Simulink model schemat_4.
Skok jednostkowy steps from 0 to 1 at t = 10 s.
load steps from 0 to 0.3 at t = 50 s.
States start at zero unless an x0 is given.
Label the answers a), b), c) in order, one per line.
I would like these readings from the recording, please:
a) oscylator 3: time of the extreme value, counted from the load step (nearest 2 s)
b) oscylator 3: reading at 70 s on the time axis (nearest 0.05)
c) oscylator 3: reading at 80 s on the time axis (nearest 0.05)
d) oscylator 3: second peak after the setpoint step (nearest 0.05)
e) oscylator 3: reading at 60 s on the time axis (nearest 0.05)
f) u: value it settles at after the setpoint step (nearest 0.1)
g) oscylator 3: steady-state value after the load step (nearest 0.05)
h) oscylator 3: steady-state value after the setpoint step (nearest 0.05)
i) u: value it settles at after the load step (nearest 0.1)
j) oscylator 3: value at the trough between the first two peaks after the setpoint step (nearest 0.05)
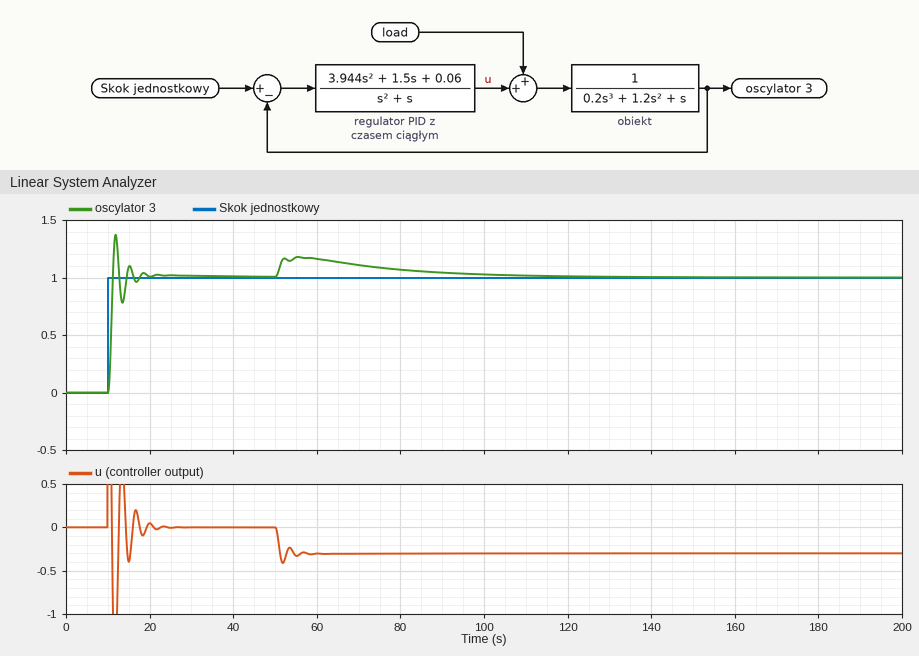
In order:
a) 6 s
b) 1.10
c) 1.05
d) 1.10
e) 1.15
f) 0.0
g) 1.00
h) 1.00
i) -0.3
j) 0.80
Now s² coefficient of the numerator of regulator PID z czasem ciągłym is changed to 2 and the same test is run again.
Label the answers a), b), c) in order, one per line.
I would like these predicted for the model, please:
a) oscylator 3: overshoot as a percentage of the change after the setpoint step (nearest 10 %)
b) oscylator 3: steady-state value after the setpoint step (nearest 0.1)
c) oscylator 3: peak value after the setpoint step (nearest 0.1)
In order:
a) 40 %
b) 1.0
c) 1.4
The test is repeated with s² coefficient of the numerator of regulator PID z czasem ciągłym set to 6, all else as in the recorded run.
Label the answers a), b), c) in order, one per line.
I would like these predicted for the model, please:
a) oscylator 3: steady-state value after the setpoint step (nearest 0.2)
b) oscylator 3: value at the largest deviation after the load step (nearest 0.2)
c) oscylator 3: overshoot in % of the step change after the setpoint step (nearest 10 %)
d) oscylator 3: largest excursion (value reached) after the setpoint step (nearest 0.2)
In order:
a) 1.0
b) 1.2
c) 50 %
d) 1.4
